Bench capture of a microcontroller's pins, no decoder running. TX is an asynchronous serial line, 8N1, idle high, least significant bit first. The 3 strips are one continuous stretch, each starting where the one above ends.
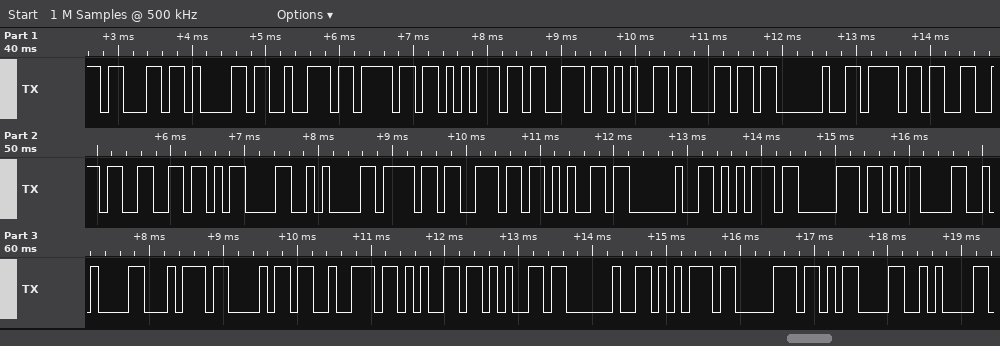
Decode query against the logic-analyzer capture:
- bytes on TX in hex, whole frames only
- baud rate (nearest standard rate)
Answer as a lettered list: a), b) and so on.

a) 0x63 0x61 0x72 0x6F 0x75 0x73 0x65 0x6C 0x20 0x6F 0x66 0x66 0x0D 0x0A 0x6F 0x6E 0x65 0x20 0x75 0x70 0x0D 0x0A 0x74 0x68 0x72 0x65 0x65 0x20 0x75 0x70 0x0D 0x0A
b) 9600 baud
